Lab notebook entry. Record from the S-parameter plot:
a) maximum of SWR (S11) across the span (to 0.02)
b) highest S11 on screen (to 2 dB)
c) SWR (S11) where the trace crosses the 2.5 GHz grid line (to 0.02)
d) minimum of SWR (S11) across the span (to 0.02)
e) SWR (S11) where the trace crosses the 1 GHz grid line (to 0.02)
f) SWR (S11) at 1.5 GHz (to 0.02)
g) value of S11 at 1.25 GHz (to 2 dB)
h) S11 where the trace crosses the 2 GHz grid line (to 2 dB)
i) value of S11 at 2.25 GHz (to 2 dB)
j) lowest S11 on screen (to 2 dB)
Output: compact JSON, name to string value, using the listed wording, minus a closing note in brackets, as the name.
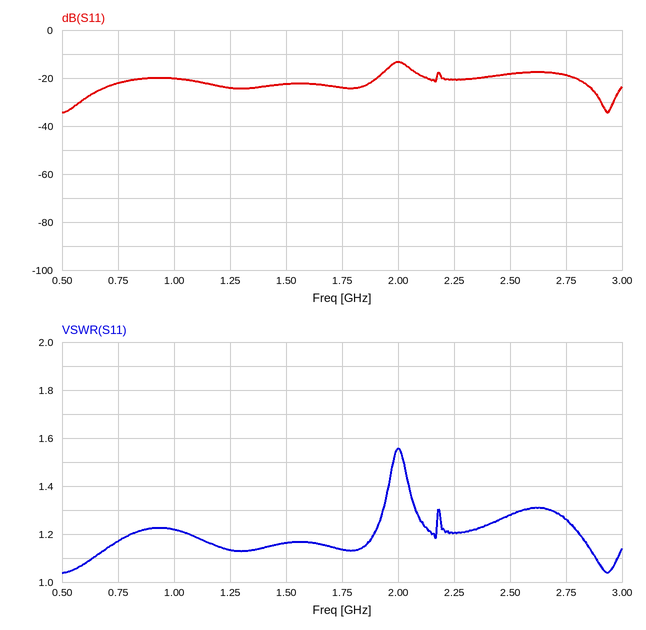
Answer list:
{"maximum of SWR (S11) across the span": "1.56", "highest S11 on screen": "-14 dB", "SWR (S11) where the trace crosses the 2.5 GHz grid line": "1.28", "minimum of SWR (S11) across the span": "1.04", "SWR (S11) where the trace crosses the 1 GHz grid line": "1.22", "SWR (S11) at 1.5 GHz": "1.16", "value of S11 at 1.25 GHz": "-24 dB", "S11 where the trace crosses the 2 GHz grid line": "-14 dB", "value of S11 at 2.25 GHz": "-20 dB", "lowest S11 on screen": "-34 dB"}
